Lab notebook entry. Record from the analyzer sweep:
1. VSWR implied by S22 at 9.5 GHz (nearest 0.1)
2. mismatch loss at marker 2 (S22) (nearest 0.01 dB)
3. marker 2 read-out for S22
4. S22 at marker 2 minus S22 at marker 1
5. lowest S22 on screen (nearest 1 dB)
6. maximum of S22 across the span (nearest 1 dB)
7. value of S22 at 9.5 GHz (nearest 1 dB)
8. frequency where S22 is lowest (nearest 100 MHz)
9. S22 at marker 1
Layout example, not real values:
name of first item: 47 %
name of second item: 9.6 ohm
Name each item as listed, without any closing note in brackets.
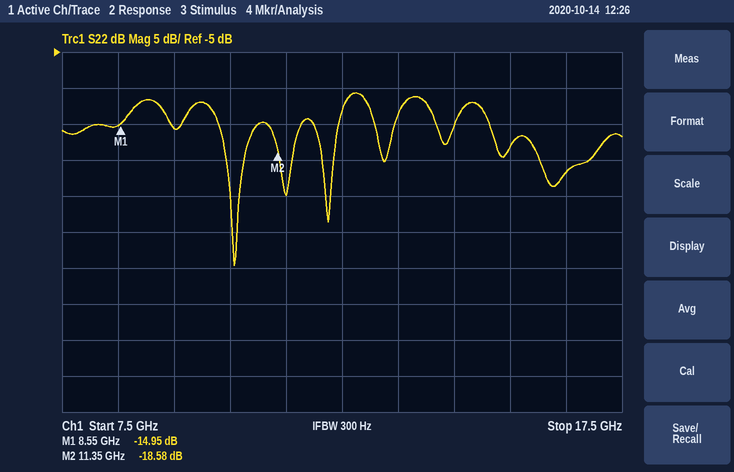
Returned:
VSWR implied by S22 at 9.5 GHz: 1.4
mismatch loss at marker 2 (S22): 0.06 dB
marker 2 read-out for S22: -18.58 dB
S22 at marker 2 minus S22 at marker 1: -3.63 dB
lowest S22 on screen: -35 dB
maximum of S22 across the span: -11 dB
value of S22 at 9.5 GHz: -16 dB
frequency where S22 is lowest: 10.6 GHz
S22 at marker 1: -14.95 dB
